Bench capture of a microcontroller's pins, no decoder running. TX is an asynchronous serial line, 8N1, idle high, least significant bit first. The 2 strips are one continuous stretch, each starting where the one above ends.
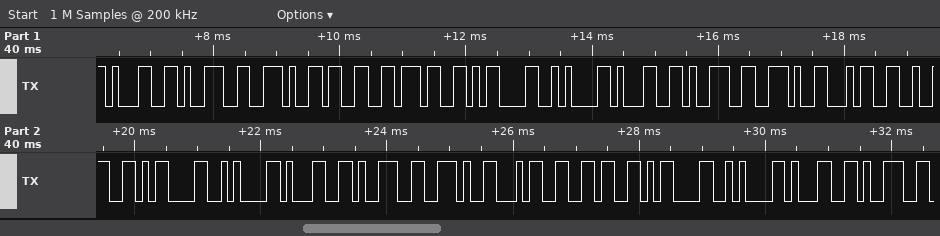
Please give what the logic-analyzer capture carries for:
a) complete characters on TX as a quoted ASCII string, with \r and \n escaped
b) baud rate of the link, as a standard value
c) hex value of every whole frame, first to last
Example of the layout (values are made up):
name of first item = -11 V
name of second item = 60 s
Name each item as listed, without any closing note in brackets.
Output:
complete characters on TX as a quoted ASCII string, with \r and \n escaped = "19.37\r\n19.42\r\n19.46\r\n19"
baud rate of the link, as a standard value = 9600 baud
hex value of every whole frame, first to last = 31 39 2E 33 37 0D 0A 31 39 2E 34 32 0D 0A 31 39 2E 34 36 0D 0A 31 39
